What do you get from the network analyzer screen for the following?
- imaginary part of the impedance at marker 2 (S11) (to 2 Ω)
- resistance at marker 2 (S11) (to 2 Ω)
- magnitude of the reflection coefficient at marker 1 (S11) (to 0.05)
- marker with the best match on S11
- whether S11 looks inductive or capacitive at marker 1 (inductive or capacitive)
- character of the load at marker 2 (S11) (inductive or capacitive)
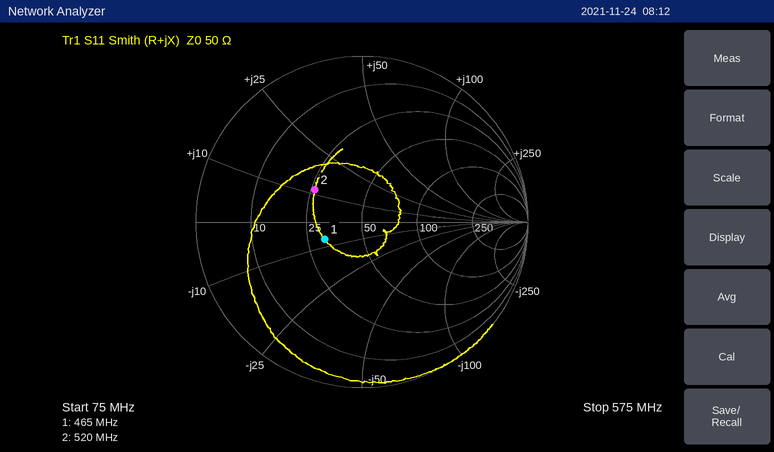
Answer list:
+12 Ω
26 Ω
0.25
marker 1
capacitive
inductive
